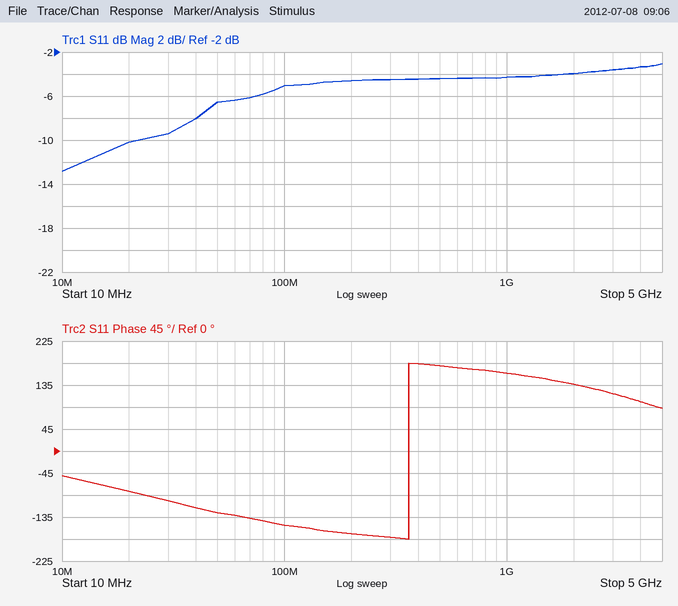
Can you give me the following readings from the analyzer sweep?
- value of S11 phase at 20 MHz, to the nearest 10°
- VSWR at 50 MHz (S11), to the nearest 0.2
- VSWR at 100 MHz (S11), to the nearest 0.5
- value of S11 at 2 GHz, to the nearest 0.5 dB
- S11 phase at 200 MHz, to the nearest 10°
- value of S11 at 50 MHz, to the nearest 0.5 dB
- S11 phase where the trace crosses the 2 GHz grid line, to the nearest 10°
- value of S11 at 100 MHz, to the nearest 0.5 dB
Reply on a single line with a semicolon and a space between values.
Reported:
-80°; 2.8; 3.5; -4.0 dB; -170°; -6.5 dB; 140°; -5.0 dB
